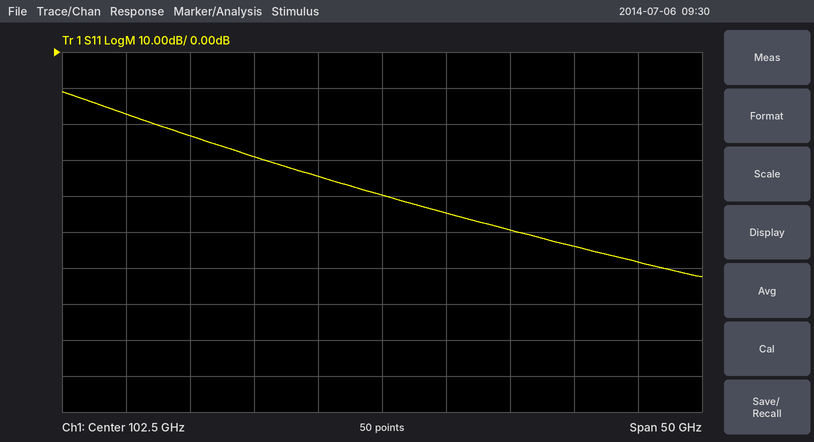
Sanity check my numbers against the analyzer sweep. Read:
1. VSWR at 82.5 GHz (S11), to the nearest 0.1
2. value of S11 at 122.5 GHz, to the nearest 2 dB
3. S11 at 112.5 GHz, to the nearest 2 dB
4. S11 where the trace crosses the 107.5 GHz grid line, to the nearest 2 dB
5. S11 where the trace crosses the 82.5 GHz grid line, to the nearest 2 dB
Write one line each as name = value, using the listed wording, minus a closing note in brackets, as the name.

VSWR at 82.5 GHz (S11), to the nearest 0.1 = 1.3
value of S11 at 122.5 GHz, to the nearest 2 dB = -58 dB
S11 at 112.5 GHz, to the nearest 2 dB = -50 dB
S11 where the trace crosses the 107.5 GHz grid line, to the nearest 2 dB = -44 dB
S11 where the trace crosses the 82.5 GHz grid line, to the nearest 2 dB = -18 dB
